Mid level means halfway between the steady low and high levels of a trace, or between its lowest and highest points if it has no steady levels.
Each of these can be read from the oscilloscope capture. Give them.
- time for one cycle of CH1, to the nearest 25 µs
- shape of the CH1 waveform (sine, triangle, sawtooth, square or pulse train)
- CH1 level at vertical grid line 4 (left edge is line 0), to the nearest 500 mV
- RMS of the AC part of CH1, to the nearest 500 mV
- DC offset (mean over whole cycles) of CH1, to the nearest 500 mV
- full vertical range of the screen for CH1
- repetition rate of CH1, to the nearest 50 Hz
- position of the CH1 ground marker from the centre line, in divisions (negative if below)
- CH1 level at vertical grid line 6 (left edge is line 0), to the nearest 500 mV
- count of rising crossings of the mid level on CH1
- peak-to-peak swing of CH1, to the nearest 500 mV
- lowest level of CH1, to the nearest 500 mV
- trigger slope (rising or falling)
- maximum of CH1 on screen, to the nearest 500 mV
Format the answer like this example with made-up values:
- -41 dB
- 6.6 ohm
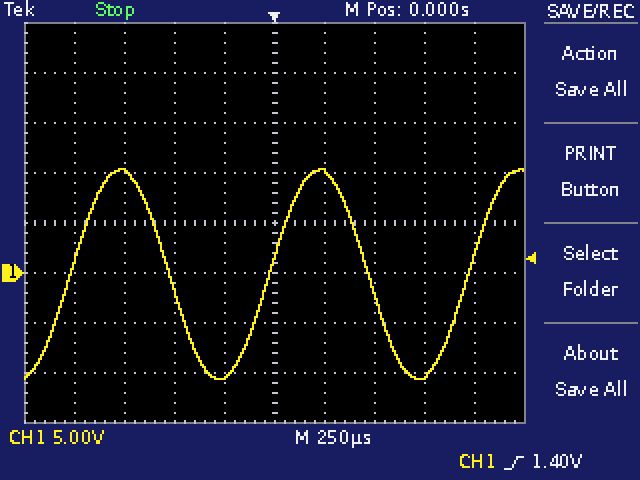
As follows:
- 1.000 ms
- sine
- -10.5 V
- 7.5 V
- 0.0 V
- 40 V
- 1.00 kHz
- -1.0 div
- 10.0 V
- 3
- 21.0 V
- -10.5 V
- rising
- 10.5 V
